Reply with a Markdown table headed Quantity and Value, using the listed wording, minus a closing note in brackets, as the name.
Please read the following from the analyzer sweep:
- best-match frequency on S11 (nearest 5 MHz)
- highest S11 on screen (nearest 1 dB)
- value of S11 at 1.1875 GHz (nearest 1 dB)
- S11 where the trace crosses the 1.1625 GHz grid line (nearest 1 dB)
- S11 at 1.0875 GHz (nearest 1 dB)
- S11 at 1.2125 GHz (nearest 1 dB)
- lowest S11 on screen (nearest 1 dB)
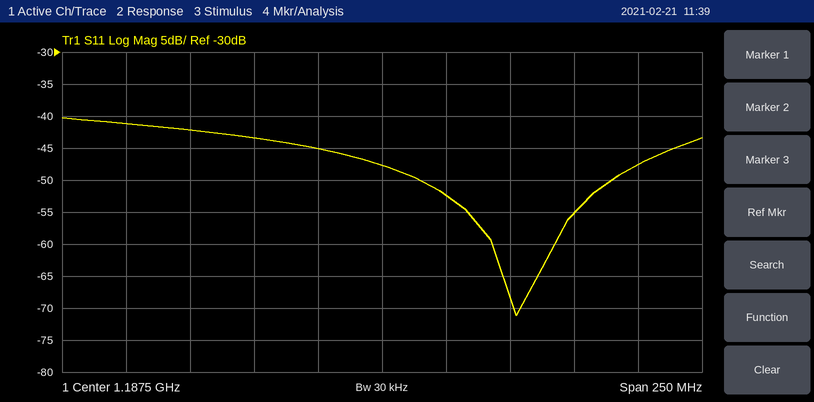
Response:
| Quantity | Value |
|---|---|
| best-match frequency on S11 | 1.240 GHz |
| highest S11 on screen | -40 dB |
| value of S11 at 1.1875 GHz | -48 dB |
| S11 where the trace crosses the 1.1625 GHz grid line | -45 dB |
| S11 at 1.0875 GHz | -41 dB |
| S11 at 1.2125 GHz | -52 dB |
| lowest S11 on screen | -71 dB |
